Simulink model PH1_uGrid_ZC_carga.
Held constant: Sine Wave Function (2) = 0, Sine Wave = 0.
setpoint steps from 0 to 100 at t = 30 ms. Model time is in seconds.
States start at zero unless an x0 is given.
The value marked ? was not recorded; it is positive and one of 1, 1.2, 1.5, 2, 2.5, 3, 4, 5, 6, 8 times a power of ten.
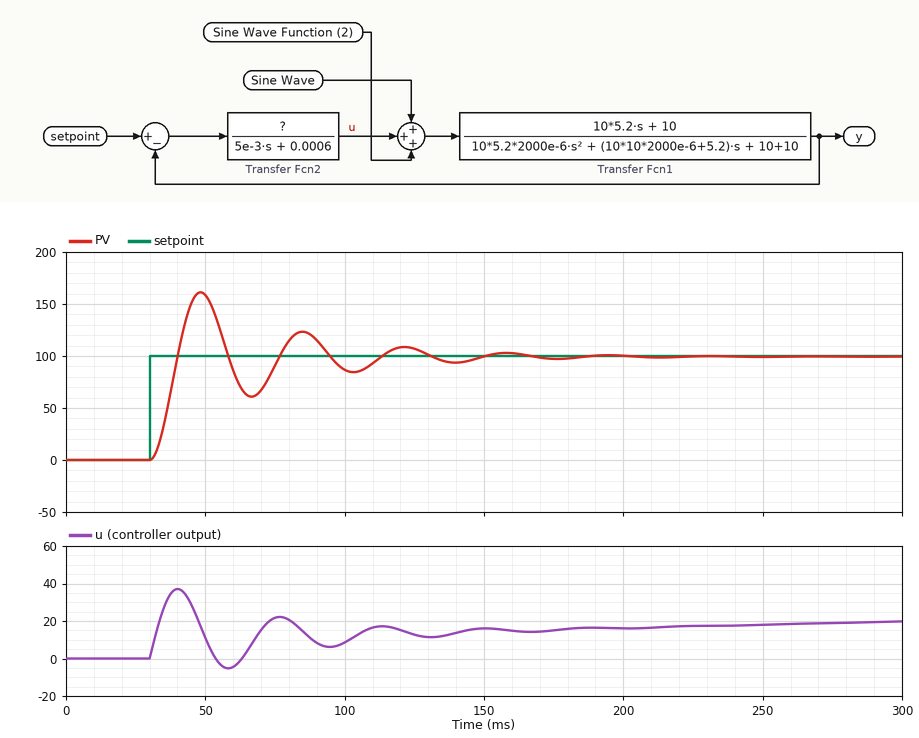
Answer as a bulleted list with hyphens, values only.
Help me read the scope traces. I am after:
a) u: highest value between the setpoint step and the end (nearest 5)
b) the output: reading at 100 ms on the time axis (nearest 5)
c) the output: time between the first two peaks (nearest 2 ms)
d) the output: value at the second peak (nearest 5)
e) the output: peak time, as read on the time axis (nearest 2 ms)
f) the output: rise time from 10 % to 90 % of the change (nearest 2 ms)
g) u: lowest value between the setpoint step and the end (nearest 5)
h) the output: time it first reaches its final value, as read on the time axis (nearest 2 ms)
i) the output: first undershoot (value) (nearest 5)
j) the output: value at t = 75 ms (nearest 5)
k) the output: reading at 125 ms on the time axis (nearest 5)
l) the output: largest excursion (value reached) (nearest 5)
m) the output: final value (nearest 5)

- 35
- 85
- 36 ms
- 125
- 48 ms
- 6 ms
- -5
- 40 ms
- 60
- 90
- 105
- 160
- 100
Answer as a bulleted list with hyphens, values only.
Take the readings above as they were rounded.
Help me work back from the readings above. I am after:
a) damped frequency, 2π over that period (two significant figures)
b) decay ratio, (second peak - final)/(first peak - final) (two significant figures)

- 0.17 rad/ms
- 0.42
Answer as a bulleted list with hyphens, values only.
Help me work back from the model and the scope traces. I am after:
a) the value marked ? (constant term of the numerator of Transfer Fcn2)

- 0.3
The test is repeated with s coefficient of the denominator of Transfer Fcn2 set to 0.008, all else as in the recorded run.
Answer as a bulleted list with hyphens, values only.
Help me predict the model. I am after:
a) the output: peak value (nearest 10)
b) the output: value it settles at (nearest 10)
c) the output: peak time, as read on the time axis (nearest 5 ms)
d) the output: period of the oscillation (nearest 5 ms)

- 150
- 100
- 55 ms
- 45 ms
